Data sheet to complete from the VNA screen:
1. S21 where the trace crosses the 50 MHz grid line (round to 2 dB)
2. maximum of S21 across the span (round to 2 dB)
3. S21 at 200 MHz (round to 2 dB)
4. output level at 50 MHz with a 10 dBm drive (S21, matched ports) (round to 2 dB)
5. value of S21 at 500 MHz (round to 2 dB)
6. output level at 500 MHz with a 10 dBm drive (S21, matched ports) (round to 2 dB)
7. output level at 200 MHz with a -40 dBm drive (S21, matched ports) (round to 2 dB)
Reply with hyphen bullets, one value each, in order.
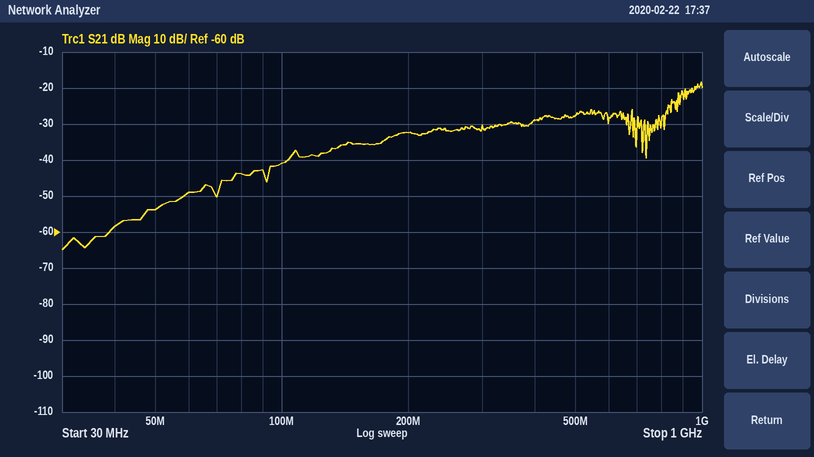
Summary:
- -54 dB
- -18 dB
- -32 dB
- -44 dBm
- -28 dB
- -18 dBm
- -72 dBm
